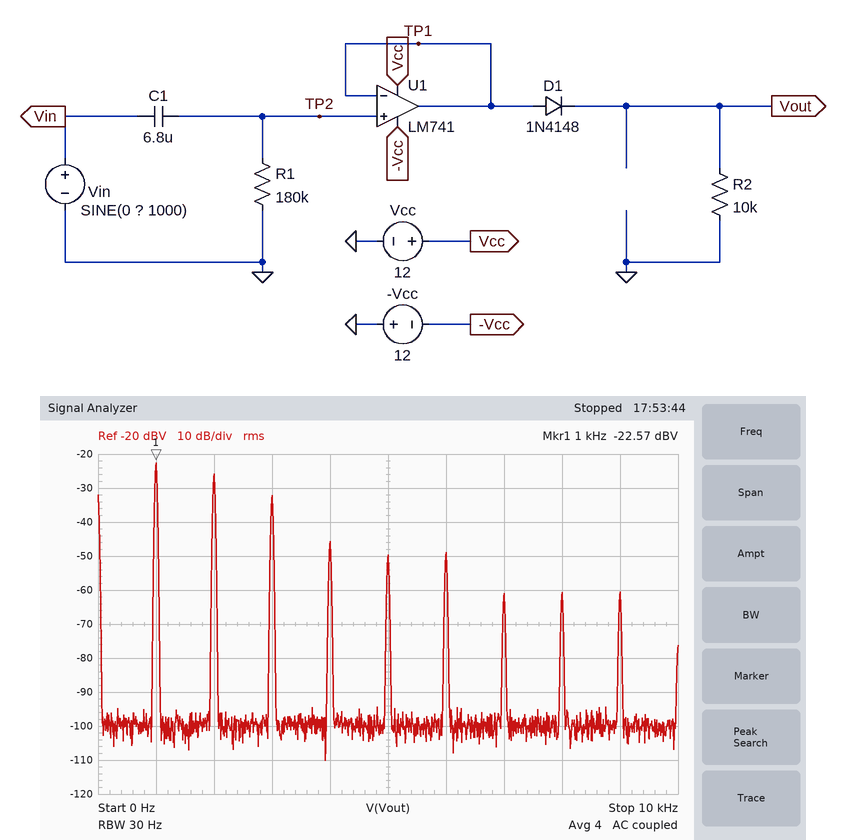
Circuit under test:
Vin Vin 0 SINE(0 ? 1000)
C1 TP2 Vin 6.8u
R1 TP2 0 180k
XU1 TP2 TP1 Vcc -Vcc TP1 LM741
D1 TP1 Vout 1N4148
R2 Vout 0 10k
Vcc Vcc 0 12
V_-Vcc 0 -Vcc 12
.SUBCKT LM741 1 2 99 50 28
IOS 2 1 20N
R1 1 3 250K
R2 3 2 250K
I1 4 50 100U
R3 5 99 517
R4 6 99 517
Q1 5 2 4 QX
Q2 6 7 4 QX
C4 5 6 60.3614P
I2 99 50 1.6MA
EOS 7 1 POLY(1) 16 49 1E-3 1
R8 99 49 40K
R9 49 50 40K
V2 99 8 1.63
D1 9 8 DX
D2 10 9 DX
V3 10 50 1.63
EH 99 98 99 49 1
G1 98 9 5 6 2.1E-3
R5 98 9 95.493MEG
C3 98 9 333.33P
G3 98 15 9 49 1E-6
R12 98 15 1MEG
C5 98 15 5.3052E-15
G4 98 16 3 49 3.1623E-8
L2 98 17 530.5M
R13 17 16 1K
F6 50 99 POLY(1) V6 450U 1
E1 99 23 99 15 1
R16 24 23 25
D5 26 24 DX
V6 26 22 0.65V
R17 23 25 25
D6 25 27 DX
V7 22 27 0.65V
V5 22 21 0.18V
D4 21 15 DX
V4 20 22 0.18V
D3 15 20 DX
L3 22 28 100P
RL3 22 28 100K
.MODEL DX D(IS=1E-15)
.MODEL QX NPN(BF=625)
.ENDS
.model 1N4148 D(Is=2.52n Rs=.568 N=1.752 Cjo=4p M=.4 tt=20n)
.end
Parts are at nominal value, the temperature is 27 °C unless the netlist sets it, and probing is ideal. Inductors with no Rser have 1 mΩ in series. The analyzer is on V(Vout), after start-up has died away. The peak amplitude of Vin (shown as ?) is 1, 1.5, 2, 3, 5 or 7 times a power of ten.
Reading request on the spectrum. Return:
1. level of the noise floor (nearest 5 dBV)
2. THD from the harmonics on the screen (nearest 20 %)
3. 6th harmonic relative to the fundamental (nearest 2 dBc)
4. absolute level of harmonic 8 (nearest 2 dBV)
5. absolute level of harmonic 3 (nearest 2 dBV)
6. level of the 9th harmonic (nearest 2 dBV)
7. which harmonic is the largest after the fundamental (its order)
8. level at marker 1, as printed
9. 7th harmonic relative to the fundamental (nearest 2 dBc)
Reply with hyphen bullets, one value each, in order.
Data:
- -100 dBV
- 80 %
- -26 dBc
- -60 dBV
- -32 dBV
- -60 dBV
- 2
- -22.57 dBV
- -38 dBc
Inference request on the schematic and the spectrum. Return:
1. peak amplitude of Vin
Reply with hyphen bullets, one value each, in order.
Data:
- 700 mV
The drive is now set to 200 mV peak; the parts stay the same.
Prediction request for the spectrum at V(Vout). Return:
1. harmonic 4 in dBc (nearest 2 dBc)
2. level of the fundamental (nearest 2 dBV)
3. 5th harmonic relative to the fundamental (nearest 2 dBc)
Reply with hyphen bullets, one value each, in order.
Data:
- -16 dBc
- -68 dBV
- -24 dBc
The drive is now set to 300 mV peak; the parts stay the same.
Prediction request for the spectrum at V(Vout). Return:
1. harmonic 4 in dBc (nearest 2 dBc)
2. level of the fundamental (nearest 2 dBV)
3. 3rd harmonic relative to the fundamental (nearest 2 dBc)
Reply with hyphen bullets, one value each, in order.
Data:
- -12 dBc
- -52 dBV
- -6 dBc
